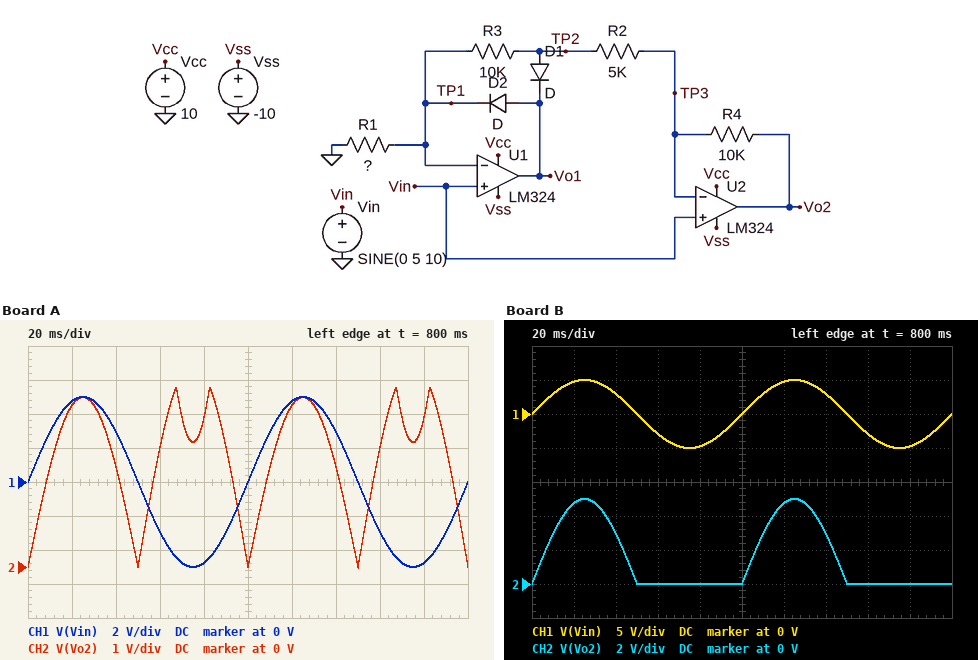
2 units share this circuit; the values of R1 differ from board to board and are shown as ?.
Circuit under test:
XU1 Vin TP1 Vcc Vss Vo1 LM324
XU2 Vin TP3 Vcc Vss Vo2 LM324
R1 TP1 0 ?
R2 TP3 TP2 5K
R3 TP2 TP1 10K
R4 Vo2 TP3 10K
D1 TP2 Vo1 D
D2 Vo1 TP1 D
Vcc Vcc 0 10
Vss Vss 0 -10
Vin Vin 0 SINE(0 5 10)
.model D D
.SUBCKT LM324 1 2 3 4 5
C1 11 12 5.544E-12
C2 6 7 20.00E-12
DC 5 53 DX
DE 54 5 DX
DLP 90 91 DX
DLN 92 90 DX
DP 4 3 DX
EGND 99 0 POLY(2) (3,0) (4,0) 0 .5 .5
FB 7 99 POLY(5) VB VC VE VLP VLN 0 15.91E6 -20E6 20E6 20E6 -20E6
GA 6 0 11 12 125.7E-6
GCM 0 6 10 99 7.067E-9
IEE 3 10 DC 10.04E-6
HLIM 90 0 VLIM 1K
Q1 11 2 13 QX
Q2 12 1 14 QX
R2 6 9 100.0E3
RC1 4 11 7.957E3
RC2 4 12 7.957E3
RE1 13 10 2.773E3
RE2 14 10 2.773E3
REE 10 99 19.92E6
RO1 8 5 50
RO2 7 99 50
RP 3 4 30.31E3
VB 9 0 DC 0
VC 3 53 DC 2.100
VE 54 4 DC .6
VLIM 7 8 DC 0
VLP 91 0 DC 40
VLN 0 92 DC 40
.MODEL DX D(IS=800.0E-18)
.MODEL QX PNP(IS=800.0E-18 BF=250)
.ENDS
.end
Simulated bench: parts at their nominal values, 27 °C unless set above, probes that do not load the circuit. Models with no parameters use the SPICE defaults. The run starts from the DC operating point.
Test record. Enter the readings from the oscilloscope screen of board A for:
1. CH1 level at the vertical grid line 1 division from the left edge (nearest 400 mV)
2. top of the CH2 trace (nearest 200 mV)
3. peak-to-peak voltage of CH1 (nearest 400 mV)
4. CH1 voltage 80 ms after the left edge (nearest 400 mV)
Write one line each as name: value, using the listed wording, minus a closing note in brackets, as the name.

CH1 level at the vertical grid line 1 division from the left edge: 4.8 V
top of the CH2 trace: 5.2 V
peak-to-peak voltage of CH1: 10.0 V
CH1 voltage 80 ms after the left edge: -4.8 V
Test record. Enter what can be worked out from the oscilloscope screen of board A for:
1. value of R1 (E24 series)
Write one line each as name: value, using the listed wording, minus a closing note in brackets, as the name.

value of R1: 9.1 kΩ
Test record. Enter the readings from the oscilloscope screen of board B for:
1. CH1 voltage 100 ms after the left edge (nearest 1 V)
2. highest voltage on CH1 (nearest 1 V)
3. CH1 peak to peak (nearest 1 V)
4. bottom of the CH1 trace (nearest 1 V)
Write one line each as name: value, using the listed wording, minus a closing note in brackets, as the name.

CH1 voltage 100 ms after the left edge: 0 V
highest voltage on CH1: 5 V
CH1 peak to peak: 10 V
bottom of the CH1 trace: -5 V
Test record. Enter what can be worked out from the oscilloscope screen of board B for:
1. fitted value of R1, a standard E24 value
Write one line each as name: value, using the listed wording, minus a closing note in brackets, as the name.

fitted value of R1, a standard E24 value: 20 kΩ
